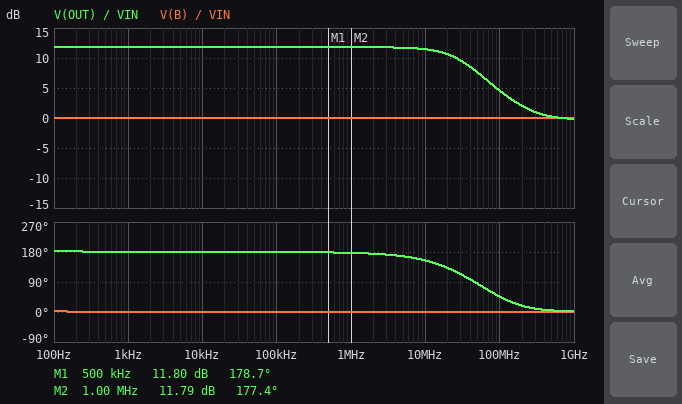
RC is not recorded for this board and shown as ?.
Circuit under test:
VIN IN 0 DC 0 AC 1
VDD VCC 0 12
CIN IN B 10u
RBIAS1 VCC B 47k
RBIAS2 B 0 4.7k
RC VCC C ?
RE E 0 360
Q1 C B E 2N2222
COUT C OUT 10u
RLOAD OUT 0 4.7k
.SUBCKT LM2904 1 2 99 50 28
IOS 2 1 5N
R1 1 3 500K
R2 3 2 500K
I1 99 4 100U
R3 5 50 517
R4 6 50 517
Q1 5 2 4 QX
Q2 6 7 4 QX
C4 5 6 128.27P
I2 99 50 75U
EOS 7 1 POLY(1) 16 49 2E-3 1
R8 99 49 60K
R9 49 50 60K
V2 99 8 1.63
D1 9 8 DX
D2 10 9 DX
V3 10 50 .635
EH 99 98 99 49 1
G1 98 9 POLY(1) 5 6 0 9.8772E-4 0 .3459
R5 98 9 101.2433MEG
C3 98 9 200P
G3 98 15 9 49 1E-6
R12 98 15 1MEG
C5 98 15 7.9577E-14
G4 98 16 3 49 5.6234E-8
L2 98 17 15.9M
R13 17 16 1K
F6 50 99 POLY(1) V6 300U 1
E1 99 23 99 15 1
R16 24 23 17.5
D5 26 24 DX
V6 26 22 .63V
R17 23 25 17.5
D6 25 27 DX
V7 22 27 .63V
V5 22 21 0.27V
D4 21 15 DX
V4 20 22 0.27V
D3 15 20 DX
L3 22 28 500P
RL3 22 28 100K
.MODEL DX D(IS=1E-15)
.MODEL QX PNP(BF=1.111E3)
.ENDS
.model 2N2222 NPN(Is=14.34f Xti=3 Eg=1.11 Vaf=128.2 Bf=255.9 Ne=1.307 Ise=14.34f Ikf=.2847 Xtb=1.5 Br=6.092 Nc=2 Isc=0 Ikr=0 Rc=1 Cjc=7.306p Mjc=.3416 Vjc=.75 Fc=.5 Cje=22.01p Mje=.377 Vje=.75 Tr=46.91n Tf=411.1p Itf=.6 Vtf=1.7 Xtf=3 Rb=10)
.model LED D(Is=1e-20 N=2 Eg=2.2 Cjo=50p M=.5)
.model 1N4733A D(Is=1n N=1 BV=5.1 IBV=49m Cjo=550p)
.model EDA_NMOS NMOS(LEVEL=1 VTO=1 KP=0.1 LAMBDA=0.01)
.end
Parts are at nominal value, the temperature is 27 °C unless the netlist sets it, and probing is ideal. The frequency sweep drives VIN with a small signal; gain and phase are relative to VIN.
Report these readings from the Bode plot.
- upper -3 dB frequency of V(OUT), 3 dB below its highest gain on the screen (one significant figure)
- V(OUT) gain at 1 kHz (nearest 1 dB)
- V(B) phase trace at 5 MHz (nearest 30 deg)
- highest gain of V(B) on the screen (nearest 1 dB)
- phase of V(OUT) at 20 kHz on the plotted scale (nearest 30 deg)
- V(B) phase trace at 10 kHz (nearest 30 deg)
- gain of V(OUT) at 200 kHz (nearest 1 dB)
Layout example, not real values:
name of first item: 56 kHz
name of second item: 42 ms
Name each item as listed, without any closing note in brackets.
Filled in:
upper -3 dB frequency of V(OUT), 3 dB below its highest gain on the screen: 40 MHz
V(OUT) gain at 1 kHz: 12 dB
V(B) phase trace at 5 MHz: 0 deg
highest gain of V(B) on the screen: 0 dB
phase of V(OUT) at 20 kHz on the plotted scale: 180 deg
V(B) phase trace at 10 kHz: 0 deg
gain of V(OUT) at 200 kHz: 12 dB
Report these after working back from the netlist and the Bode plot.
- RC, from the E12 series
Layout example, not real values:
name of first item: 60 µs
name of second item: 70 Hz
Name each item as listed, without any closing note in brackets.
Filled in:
RC, from the E12 series: 2.2 kΩ
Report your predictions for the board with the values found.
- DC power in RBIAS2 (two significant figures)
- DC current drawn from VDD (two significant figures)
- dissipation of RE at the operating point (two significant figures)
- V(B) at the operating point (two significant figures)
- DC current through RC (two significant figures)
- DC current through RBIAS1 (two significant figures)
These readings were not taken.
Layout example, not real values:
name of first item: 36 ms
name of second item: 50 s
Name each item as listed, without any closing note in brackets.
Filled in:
DC power in RBIAS2: 240 µW
DC current drawn from VDD: 1.4 mA
dissipation of RE at the operating point: 470 µW
V(B) at the operating point: 1.1 V
DC current through RC: 1.1 mA
DC current through RBIAS1: 230 µA
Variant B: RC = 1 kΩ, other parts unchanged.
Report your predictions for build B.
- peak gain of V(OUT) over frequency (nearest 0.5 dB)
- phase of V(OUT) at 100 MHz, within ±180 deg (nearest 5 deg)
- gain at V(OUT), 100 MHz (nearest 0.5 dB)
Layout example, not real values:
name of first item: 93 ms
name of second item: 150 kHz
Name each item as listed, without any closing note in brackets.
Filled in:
peak gain of V(OUT) over frequency: 6.5 dB
phase of V(OUT) at 100 MHz, within ±180 deg: 60 deg
gain at V(OUT), 100 MHz: 3.5 dB
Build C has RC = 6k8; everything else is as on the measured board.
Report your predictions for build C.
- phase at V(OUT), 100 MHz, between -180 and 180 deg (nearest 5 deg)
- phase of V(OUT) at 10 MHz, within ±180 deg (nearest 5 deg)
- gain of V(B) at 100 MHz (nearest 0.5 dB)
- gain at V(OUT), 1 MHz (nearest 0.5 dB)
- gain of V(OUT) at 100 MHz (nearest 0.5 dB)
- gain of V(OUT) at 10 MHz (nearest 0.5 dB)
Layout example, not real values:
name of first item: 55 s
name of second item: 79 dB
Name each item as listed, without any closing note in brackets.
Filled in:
phase at V(OUT), 100 MHz, between -180 and 180 deg: 30 deg
phase of V(OUT) at 10 MHz, within ±180 deg: 135 deg
gain of V(B) at 100 MHz: 0 dB
gain at V(OUT), 1 MHz: 17.0 dB
gain of V(OUT) at 100 MHz: 4.0 dB
gain of V(OUT) at 10 MHz: 15.5 dB
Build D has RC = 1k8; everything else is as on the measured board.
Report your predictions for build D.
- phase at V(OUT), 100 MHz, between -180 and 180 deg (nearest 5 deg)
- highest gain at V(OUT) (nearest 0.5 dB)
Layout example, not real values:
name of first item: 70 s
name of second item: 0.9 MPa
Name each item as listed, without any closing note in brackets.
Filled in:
phase at V(OUT), 100 MHz, between -180 and 180 deg: 50 deg
highest gain at V(OUT): 10.5 dB
